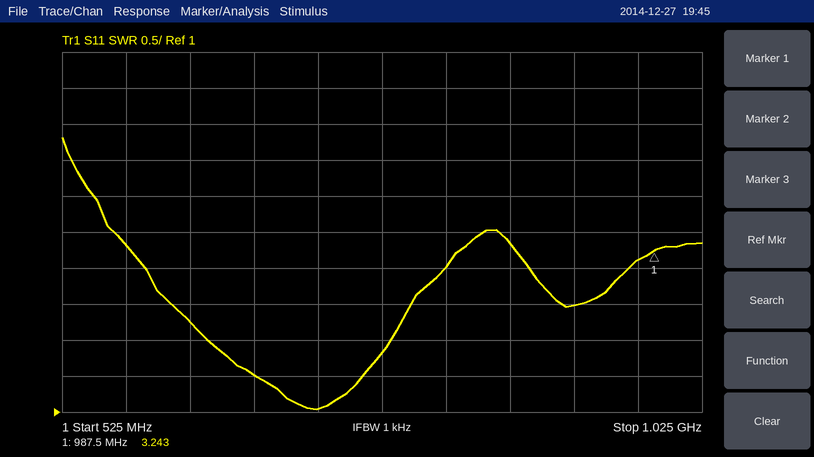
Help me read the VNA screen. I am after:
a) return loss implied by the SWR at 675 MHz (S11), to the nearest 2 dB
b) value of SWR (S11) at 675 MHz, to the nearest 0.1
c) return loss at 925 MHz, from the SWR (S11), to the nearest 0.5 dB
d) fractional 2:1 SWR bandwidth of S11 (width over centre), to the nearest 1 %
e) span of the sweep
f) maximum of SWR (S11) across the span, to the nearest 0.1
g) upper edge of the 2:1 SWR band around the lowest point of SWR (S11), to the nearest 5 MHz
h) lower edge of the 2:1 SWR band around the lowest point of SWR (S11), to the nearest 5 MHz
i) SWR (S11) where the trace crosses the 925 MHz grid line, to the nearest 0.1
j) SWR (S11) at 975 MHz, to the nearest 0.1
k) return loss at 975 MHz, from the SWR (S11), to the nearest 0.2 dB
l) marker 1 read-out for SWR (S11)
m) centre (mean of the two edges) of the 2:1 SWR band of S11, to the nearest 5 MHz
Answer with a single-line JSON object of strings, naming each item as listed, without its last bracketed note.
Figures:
{"return loss implied by the SWR at 675 MHz (S11), to the nearest 2 dB": "14 dB", "value of SWR (S11) at 675 MHz, to the nearest 0.1": "1.5", "return loss at 925 MHz, from the SWR (S11), to the nearest 0.5 dB": "7.5 dB", "fractional 2:1 SWR bandwidth of S11 (width over centre), to the nearest 1 %": "20 %", "span of the sweep": "500 MHz", "maximum of SWR (S11) across the span, to the nearest 0.1": "4.8", "upper edge of the 2:1 SWR band around the lowest point of SWR (S11), to the nearest 5 MHz": "780 MHz", "lower edge of the 2:1 SWR band around the lowest point of SWR (S11), to the nearest 5 MHz": "640 MHz", "SWR (S11) where the trace crosses the 925 MHz grid line, to the nearest 0.1": "2.5", "SWR (S11) at 975 MHz, to the nearest 0.1": "3.1", "return loss at 975 MHz, from the SWR (S11), to the nearest 0.2 dB": "5.8 dB", "marker 1 read-out for SWR": "3.243", "centre (mean of the two edges) of the 2:1 SWR band of S11, to the nearest 5 MHz": "710 MHz"}
